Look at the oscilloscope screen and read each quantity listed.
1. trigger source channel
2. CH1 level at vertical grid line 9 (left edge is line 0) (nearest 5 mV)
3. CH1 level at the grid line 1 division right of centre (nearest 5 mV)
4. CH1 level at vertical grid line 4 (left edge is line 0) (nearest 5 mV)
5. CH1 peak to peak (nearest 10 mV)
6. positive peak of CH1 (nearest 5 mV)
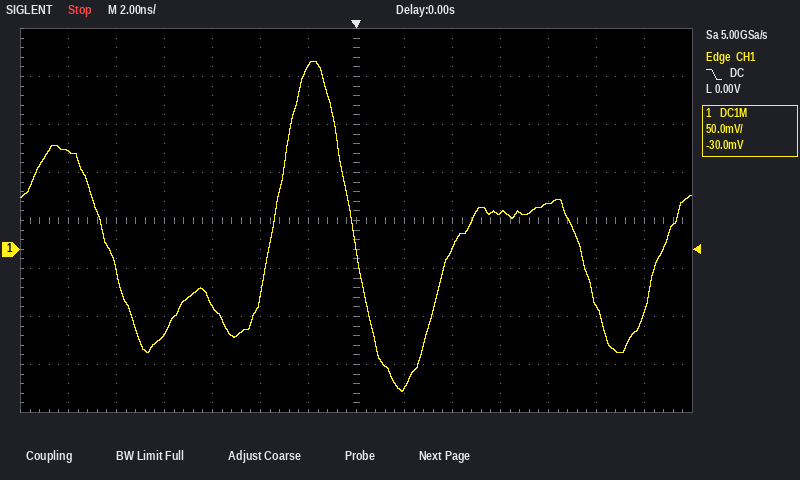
CH1
0 mV
-145 mV
-60 mV
340 mV
195 mV
